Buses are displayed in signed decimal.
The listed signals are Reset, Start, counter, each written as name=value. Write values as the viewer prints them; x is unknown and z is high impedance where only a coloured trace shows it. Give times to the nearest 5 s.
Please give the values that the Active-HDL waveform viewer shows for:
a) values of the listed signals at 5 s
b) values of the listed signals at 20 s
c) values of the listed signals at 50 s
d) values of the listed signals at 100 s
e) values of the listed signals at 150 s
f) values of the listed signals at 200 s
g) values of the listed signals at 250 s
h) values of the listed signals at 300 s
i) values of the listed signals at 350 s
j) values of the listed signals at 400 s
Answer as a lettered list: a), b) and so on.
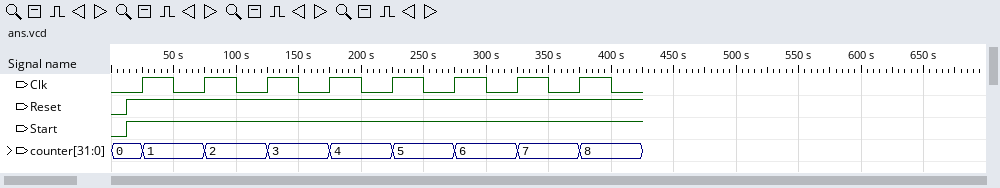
a) Reset=0, Start=0, counter=0
b) Reset=1, Start=1, counter=0
c) Reset=1, Start=1, counter=1
d) Reset=1, Start=1, counter=2
e) Reset=1, Start=1, counter=3
f) Reset=1, Start=1, counter=4
g) Reset=1, Start=1, counter=5
h) Reset=1, Start=1, counter=6
i) Reset=1, Start=1, counter=7
j) Reset=1, Start=1, counter=8
